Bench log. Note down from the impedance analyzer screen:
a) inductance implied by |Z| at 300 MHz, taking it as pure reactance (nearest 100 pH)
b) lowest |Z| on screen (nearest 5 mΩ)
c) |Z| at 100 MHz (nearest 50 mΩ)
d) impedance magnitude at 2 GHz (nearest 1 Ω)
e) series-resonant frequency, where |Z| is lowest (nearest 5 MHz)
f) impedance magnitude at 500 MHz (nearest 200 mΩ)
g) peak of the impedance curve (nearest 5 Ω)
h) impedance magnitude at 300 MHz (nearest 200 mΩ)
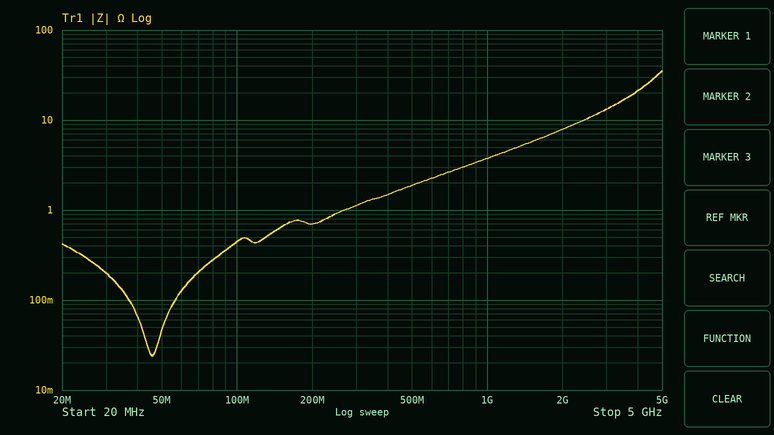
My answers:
600 pH
25 mΩ
450 mΩ
8 Ω
45 MHz
1.8 Ω
35 Ω
1.2 Ω
